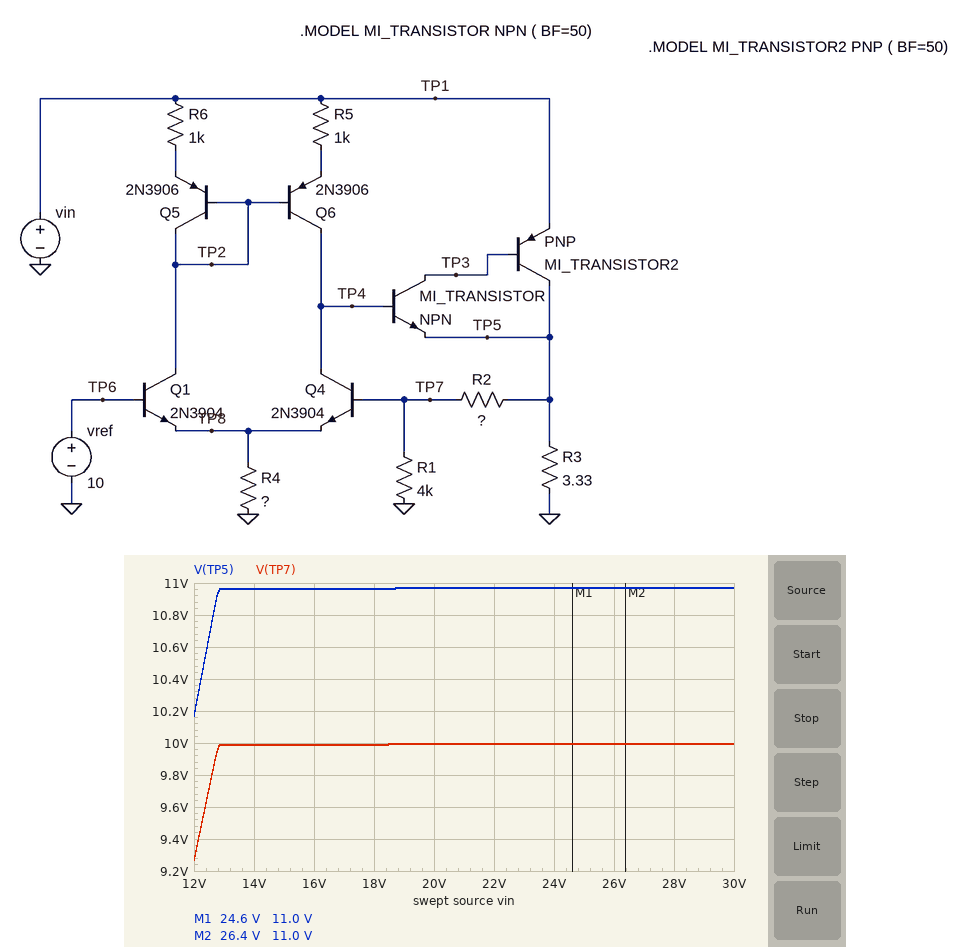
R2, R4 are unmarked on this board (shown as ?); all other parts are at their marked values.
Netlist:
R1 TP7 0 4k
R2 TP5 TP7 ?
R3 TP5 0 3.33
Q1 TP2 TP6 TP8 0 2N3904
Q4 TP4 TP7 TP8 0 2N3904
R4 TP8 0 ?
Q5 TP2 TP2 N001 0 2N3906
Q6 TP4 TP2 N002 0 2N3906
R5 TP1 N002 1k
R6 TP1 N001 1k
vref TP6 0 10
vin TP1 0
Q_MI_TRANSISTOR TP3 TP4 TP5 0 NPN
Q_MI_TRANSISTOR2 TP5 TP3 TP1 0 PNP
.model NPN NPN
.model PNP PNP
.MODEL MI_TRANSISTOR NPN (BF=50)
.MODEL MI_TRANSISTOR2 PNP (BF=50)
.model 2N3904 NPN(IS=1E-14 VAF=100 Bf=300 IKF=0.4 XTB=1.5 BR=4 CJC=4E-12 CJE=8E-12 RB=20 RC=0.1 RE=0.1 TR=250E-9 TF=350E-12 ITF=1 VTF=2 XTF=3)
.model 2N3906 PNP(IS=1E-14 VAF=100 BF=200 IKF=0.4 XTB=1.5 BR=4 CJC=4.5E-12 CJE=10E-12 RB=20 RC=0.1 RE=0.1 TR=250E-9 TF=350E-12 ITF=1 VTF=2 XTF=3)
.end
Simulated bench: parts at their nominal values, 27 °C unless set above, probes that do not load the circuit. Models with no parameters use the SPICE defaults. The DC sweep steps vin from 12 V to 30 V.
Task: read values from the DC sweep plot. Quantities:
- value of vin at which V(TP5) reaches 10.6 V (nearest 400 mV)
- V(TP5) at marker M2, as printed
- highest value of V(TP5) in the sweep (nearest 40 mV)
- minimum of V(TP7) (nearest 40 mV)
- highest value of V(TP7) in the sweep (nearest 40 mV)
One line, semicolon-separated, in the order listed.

12.4 V; 11.0 V; 10.96 V; 9.28 V; 10.00 V
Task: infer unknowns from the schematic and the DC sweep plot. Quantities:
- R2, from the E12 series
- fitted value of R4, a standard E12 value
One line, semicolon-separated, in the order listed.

390 Ω; 5.6 kΩ
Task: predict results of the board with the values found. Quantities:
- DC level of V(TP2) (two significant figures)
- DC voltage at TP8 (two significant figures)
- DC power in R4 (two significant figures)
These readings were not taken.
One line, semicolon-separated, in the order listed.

9.3 V; 9.3 V; 15 mW
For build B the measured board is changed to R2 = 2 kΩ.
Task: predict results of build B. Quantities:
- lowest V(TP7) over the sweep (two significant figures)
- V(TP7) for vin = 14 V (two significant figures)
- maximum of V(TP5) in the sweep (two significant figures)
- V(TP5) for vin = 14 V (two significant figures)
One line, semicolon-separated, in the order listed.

6.8 V; 8.1 V; 15 V; 12 V
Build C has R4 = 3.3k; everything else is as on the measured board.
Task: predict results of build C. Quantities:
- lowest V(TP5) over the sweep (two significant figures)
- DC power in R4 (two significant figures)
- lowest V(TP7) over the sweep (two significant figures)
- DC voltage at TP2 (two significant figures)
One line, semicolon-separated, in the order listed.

9.6 V; 26 mW; 8.8 V; 9.2 V
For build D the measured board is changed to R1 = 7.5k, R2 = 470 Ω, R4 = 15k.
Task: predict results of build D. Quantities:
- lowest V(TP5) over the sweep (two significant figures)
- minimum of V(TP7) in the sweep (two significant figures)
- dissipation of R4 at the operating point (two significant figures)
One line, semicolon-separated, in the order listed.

11 V; 10 V; 5.8 mW
